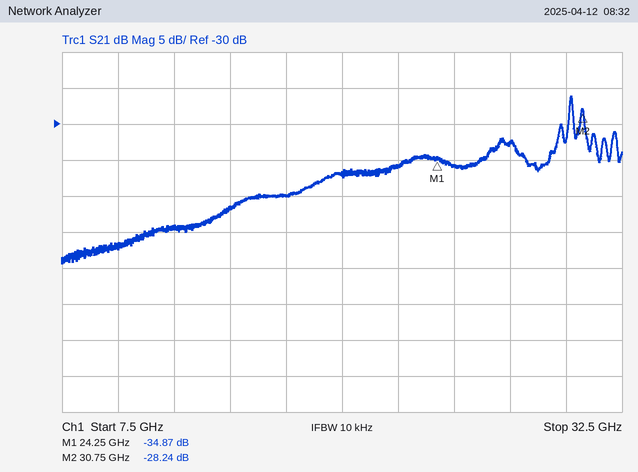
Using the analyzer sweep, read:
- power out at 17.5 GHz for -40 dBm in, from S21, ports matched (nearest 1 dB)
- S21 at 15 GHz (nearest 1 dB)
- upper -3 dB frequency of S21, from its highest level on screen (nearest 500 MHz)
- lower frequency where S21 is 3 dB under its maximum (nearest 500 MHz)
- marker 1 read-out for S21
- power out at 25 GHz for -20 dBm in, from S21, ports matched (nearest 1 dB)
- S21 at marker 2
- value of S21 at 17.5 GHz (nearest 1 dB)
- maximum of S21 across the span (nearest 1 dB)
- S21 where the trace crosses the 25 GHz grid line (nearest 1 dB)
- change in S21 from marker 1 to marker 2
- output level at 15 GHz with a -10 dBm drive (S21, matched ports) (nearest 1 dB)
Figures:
-80 dBm
-42 dB
30.5 GHz
30.0 GHz
-34.87 dB
-56 dBm
-28.24 dB
-40 dB
-26 dB
-36 dB
6.63 dB
-52 dBm
